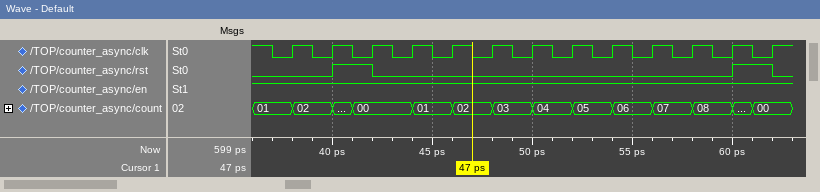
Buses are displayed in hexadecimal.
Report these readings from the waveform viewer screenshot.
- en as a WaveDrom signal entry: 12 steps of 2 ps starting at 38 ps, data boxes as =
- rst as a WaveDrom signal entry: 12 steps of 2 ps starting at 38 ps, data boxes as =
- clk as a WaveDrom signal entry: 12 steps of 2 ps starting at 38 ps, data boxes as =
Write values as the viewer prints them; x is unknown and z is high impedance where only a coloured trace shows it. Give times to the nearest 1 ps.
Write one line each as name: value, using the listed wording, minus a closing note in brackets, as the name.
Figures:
en as a WaveDrom signal entry: 12 steps of 2 ps starting at 38 ps, data boxes as =: {name: 'en', wave: '1...........'}
rst as a WaveDrom signal entry: 12 steps of 2 ps starting at 38 ps, data boxes as =: {name: 'rst', wave: '010........1'}
clk as a WaveDrom signal entry: 12 steps of 2 ps starting at 38 ps, data boxes as =: {name: 'clk', wave: 'p...........'}
